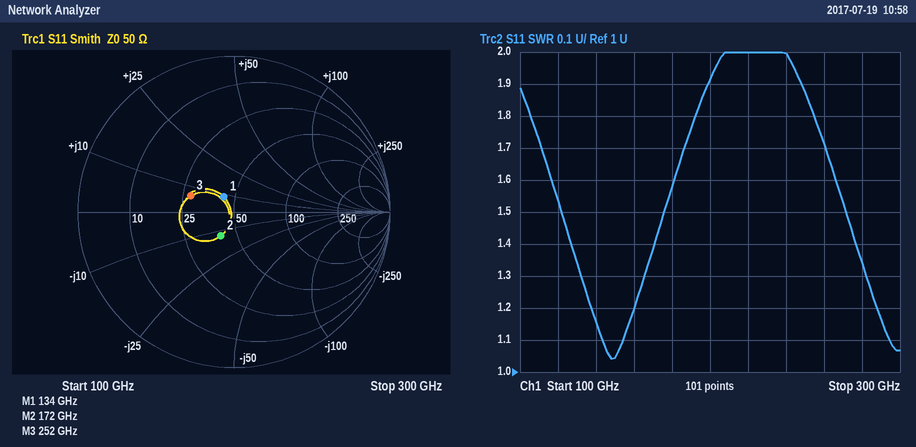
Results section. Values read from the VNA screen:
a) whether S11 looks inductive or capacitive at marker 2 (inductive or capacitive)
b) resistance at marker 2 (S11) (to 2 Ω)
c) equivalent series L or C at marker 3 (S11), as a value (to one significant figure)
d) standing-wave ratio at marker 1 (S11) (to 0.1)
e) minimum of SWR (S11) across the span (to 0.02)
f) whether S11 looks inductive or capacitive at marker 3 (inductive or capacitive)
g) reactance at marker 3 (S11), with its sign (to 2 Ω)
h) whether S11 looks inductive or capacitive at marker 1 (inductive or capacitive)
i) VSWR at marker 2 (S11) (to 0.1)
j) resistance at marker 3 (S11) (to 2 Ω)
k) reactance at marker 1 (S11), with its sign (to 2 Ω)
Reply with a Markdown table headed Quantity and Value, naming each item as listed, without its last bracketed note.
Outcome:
| Quantity | Value |
|---|---|
| whether S11 looks inductive or capacitive at marker 2 | capacitive |
| resistance at marker 2 (S11) | 40 Ω |
| equivalent series L or C at marker 3 (S11), as a value | 4 pH |
| standing-wave ratio at marker 1 (S11) | 1.3 |
| minimum of SWR (S11) across the span | 1.04 |
| whether S11 looks inductive or capacitive at marker 3 | inductive |
| reactance at marker 3 (S11), with its sign | +6 Ω |
| whether S11 looks inductive or capacitive at marker 1 | inductive |
| VSWR at marker 2 (S11) | 1.4 |
| resistance at marker 3 (S11) | 28 Ω |
| reactance at marker 1 (S11), with its sign | +8 Ω |
